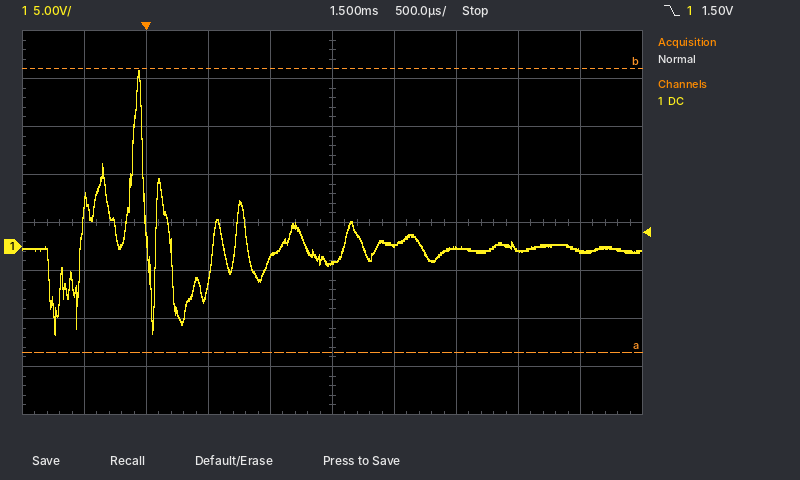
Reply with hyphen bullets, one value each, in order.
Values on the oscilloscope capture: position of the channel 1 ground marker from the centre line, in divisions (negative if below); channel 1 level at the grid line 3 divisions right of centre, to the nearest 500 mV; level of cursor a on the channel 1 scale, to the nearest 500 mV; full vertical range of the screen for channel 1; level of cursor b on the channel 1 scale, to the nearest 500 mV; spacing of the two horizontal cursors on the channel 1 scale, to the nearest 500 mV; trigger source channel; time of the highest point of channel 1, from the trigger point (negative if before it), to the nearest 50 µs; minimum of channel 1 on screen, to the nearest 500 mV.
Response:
- -0.5 div
- -500 mV
- -11.0 V
- 40 V
- 18.5 V
- 29.5 V
- channel 1
- -50 µs
- -9.0 V
